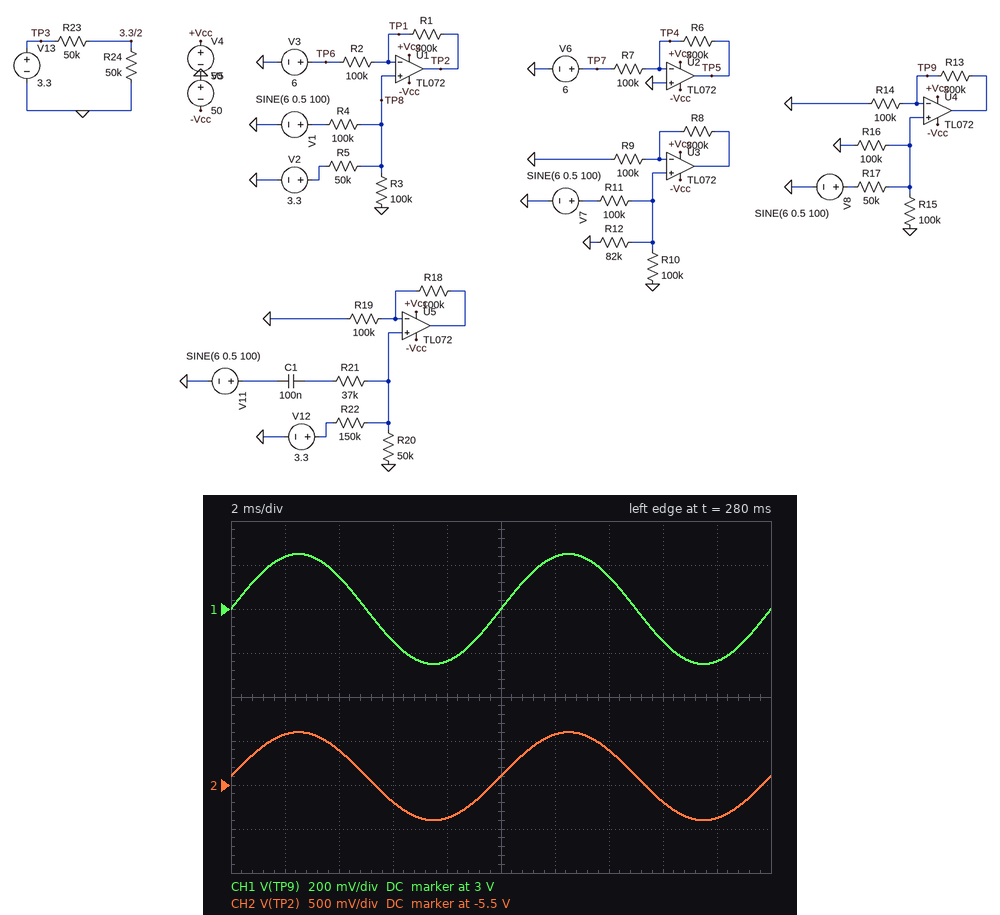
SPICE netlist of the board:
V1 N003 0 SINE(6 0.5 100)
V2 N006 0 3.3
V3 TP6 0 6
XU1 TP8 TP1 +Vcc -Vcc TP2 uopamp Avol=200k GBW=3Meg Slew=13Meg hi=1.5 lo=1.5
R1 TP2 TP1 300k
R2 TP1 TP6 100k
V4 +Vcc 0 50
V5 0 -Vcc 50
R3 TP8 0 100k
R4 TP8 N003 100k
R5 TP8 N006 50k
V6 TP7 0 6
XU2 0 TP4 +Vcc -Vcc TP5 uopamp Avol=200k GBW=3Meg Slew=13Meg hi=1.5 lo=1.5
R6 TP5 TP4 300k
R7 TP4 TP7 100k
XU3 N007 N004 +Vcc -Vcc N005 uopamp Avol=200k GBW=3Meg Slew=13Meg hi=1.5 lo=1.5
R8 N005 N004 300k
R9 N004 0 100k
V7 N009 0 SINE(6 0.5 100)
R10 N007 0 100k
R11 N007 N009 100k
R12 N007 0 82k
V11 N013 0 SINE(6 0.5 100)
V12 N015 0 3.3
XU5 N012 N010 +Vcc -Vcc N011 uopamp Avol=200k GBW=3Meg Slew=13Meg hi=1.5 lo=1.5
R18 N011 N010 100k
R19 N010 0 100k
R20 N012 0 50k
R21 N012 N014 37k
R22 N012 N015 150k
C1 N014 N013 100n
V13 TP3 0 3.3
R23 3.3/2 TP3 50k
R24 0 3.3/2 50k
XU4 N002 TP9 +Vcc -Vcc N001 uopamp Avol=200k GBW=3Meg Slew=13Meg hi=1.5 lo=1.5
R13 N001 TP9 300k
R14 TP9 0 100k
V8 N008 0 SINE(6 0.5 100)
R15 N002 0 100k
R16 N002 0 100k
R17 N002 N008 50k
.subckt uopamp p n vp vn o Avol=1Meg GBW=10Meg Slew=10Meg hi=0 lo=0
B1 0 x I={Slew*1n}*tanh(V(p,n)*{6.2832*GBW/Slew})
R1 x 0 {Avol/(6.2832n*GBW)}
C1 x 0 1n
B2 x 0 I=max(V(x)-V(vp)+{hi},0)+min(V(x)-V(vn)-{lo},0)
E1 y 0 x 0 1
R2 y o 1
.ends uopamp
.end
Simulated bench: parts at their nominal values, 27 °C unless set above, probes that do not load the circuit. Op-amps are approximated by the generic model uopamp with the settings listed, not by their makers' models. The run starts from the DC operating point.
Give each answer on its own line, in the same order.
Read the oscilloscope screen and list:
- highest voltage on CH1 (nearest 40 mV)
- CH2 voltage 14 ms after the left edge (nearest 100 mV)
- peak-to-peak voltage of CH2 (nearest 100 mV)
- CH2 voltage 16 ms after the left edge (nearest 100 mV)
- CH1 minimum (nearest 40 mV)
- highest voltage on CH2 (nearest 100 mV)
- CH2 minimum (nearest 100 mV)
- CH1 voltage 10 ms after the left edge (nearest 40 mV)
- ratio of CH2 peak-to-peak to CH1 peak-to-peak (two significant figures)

3.24 V
-5.1 V
1.0 V
-5.7 V
2.76 V
-4.9 V
-5.9 V
3.00 V
2.0
